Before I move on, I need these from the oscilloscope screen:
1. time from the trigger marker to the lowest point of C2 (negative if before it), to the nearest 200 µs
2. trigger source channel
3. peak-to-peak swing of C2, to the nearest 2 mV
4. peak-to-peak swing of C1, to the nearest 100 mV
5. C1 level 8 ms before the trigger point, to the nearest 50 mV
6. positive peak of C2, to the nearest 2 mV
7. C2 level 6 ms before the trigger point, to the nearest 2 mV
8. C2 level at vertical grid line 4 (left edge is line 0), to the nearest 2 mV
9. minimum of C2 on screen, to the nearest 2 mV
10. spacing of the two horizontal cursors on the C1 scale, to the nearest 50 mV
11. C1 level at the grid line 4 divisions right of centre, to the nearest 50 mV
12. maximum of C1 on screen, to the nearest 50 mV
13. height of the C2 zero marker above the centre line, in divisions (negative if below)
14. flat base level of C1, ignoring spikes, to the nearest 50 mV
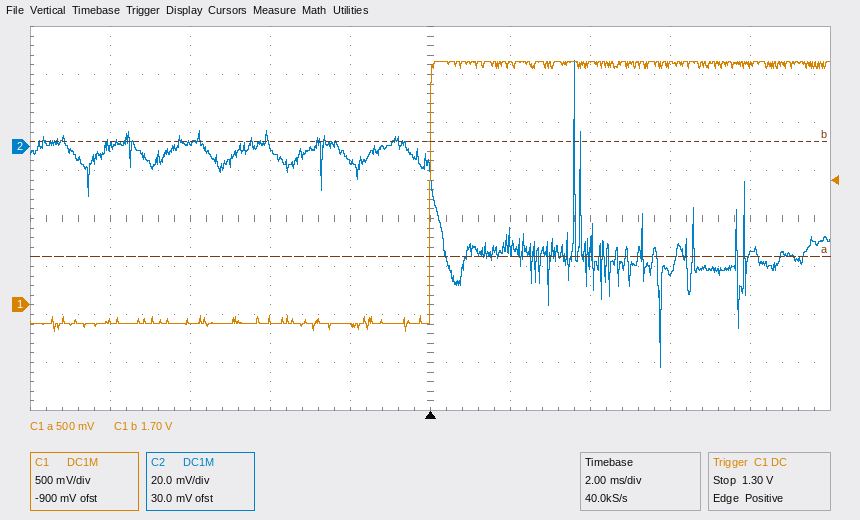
+5.8 ms
C1
128 mV
2.80 V
-150 mV
36 mV
2 mV
-6 mV
-92 mV
1.20 V
2.50 V
2.55 V
+1.5 div
-200 mV
